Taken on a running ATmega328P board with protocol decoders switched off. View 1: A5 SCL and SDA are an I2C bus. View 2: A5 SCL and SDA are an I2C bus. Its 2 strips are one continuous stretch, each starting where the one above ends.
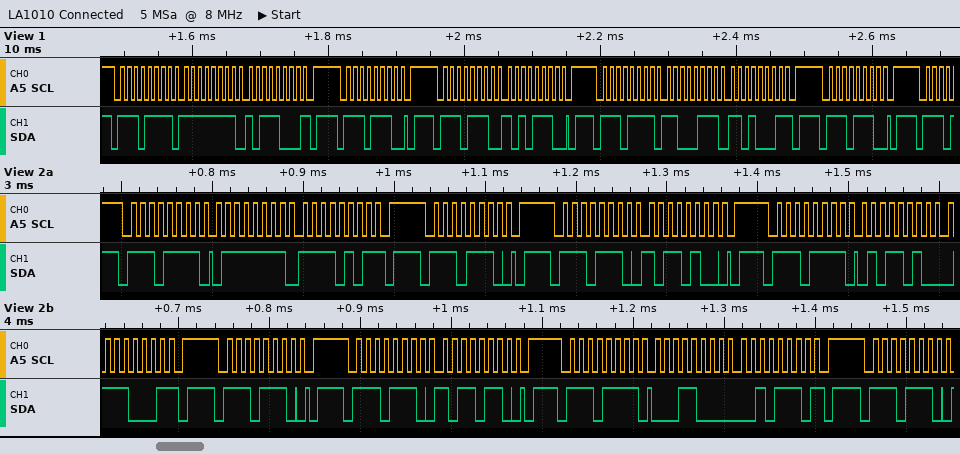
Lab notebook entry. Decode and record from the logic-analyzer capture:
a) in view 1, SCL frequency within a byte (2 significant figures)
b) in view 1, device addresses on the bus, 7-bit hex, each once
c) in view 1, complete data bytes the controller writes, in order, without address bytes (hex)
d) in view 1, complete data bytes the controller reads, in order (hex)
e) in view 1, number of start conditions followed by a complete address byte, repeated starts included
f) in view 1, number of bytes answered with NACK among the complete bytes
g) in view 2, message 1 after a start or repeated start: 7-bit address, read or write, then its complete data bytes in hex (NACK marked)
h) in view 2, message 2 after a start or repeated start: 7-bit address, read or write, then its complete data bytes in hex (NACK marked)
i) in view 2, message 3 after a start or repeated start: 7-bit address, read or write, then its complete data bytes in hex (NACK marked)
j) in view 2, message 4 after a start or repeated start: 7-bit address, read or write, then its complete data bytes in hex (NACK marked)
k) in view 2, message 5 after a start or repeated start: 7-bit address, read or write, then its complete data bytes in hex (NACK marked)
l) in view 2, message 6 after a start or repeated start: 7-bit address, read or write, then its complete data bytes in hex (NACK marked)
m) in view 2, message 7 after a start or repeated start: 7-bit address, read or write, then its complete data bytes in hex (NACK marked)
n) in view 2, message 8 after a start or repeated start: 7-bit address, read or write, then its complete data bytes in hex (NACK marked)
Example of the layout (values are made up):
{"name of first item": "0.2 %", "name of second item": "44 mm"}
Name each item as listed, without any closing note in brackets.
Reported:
{"in view 1, SCL frequency within a byte": "100 kHz", "in view 1, device addresses on the bus, 7-bit hex, each once": "0x77", "in view 1, complete data bytes the controller writes, in order, without address bytes": "AE", "in view 1, complete data bytes the controller reads, in order": "FF B8 C7 D1", "in view 1, number of start conditions followed by a complete address byte, repeated starts included": "5", "in view 1, number of bytes answered with NACK among the complete bytes": "2", "in view 2, message 1 after a start or repeated start: 7-bit address, read or write, then its complete data bytes in hex": "0x77 read: 7F F5 NACK", "in view 2, message 2 after a start or repeated start: 7-bit address, read or write, then its complete data bytes in hex": "0x77 write", "in view 2, message 3 after a start or repeated start: 7-bit address, read or write, then its complete data bytes in hex": "0x77 write: B4", "in view 2, message 4 after a start or repeated start: 7-bit address, read or write, then its complete data bytes in hex": "0x77 read: 5A 71 NACK", "in view 2, message 5 after a start or repeated start: 7-bit address, read or write, then its complete data bytes in hex": "0x77 write", "in view 2, message 6 after a start or repeated start: 7-bit address, read or write, then its complete data bytes in hex": "0x77 write: B6", "in view 2, message 7 after a start or repeated start: 7-bit address, read or write, then its complete data bytes in hex": "0x77 read: 18 2E NACK", "in view 2, message 8 after a start or repeated start: 7-bit address, read or write, then its complete data bytes in hex": "0x77 write"}
